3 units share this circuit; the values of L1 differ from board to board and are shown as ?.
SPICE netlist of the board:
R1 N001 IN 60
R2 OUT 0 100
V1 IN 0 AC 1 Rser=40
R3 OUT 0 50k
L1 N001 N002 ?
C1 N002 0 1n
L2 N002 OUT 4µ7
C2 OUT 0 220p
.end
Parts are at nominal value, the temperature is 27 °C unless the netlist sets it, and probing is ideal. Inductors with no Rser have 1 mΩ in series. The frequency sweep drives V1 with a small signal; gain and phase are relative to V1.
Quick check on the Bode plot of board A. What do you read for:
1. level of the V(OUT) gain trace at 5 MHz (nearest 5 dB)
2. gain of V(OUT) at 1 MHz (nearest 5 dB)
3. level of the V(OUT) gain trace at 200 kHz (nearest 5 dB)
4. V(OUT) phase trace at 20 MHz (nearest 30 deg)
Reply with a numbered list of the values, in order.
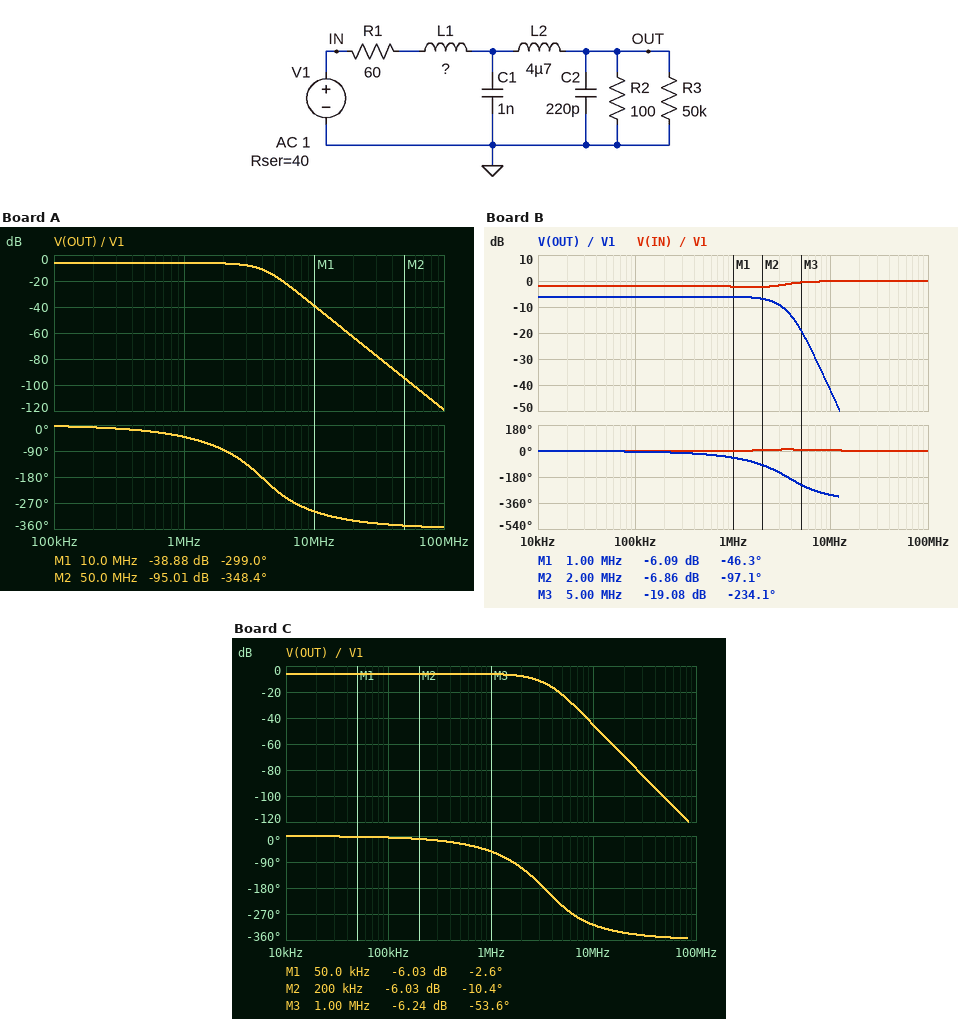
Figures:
1. -15 dB
2. -5 dB
3. -5 dB
4. -330 deg
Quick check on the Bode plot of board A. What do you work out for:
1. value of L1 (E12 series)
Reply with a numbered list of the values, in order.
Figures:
1. 5.6 µH
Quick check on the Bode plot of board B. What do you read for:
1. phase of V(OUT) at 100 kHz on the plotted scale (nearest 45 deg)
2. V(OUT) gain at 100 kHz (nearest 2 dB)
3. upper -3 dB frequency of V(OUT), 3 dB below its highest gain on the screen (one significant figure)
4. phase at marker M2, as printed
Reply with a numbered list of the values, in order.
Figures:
1. 0 deg
2. -6 dB
3. 3 MHz
4. -97.1 deg
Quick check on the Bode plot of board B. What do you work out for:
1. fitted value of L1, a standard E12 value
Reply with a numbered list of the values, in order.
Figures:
1. 8.2 µH
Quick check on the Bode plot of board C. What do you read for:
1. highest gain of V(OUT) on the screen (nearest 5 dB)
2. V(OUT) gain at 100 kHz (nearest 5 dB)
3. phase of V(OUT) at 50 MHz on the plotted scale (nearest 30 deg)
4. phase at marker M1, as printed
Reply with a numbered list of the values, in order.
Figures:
1. -5 dB
2. -5 dB
3. -360 deg
4. -2.6 deg
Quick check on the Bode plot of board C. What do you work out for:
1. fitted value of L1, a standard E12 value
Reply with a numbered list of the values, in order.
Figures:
1. 12 µH
